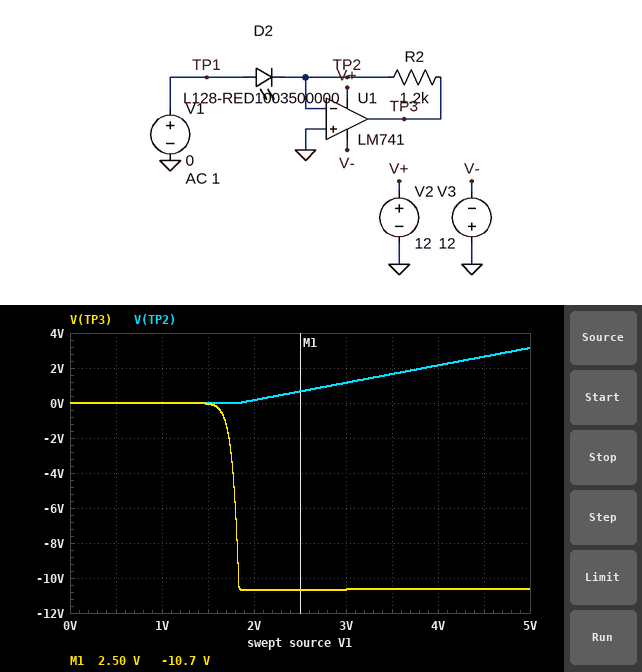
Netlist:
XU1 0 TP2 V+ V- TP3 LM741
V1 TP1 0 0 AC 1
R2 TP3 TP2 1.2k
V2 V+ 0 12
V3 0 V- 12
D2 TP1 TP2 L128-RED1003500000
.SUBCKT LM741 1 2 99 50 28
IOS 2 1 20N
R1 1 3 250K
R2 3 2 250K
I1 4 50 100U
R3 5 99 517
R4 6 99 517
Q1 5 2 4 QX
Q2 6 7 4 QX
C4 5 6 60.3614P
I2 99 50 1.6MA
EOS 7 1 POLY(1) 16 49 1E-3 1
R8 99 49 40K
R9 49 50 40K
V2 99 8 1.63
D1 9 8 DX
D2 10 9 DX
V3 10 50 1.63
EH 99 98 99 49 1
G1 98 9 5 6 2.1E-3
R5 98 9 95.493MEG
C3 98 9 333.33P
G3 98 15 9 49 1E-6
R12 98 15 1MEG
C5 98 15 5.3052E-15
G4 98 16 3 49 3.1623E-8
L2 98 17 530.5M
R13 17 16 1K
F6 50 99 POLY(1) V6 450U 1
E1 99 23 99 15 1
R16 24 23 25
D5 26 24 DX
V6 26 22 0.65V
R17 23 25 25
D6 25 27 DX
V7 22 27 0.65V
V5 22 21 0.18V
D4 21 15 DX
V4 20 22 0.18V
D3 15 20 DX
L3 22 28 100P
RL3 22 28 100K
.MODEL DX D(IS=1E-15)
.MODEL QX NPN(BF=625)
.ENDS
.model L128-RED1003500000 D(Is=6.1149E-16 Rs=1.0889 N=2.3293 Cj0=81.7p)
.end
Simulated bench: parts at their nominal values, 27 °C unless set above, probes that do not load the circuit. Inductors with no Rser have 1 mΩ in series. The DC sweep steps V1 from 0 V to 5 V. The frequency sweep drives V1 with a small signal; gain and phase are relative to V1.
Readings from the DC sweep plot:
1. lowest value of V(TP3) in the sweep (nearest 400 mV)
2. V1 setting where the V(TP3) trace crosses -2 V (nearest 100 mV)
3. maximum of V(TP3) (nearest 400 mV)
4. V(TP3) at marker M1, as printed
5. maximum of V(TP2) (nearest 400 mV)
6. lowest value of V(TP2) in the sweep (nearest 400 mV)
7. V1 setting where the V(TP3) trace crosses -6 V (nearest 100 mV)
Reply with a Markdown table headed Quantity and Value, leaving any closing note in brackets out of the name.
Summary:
| Quantity | Value |
|---|---|
| lowest value of V(TP3) in the sweep | -10.8 V |
| V1 setting where the V(TP3) trace crosses -2 V | 1.7 V |
| maximum of V(TP3) | 0 V |
| V(TP3) at marker M1, as printed | -10.7 V |
| maximum of V(TP2) | 3.2 V |
| lowest value of V(TP2) in the sweep | 0 V |
| V1 setting where the V(TP3) trace crosses -6 V | 1.8 V |
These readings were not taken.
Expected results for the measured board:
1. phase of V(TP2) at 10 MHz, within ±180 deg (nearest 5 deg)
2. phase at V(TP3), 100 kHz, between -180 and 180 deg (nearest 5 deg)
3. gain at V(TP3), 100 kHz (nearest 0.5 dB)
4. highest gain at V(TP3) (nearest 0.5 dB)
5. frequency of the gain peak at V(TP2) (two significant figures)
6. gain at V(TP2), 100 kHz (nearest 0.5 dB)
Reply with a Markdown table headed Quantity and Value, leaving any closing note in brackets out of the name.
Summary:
| Quantity | Value |
|---|---|
| phase of V(TP2) at 10 MHz, within ±180 deg | 10 deg |
| phase at V(TP3), 100 kHz, between -180 and 180 deg | -95 deg |
| gain at V(TP3), 100 kHz | -24.0 dB |
| highest gain at V(TP3) | 0.5 dB |
| frequency of the gain peak at V(TP2) | 1.2 MHz |
| gain at V(TP2), 100 kHz | -43.0 dB |
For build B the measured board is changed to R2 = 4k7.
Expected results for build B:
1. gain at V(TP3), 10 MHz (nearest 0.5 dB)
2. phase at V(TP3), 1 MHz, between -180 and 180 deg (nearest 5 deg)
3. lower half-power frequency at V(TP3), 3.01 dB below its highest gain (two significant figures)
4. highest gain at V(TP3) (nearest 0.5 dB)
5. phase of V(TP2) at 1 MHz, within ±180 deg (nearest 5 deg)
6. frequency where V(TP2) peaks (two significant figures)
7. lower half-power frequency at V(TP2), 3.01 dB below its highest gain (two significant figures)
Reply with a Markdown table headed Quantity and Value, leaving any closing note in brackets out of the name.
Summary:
| Quantity | Value |
|---|---|
| gain at V(TP3), 10 MHz | -24.5 dB |
| phase at V(TP3), 1 MHz, between -180 and 180 deg | 80 deg |
| lower half-power frequency at V(TP3), 3.01 dB below its highest gain | 510 kHz |
| highest gain at V(TP3) | 12.5 dB |
| phase of V(TP2) at 1 MHz, within ±180 deg | 20 deg |
| frequency where V(TP2) peaks | 630 kHz |
| lower half-power frequency at V(TP2), 3.01 dB below its highest gain | 540 kHz |
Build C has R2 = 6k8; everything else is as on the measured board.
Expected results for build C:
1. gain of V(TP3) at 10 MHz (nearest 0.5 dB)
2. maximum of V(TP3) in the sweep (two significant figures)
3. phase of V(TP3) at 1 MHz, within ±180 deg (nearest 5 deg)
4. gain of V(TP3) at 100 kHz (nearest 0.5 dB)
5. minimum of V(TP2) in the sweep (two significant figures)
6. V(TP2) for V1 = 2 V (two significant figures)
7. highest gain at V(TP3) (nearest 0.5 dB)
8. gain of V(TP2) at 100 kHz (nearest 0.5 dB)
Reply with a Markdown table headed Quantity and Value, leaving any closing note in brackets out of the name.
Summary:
| Quantity | Value |
|---|---|
| gain of V(TP3) at 10 MHz | -26.0 dB |
| maximum of V(TP3) in the sweep | 1.7 mV |
| phase of V(TP3) at 1 MHz, within ±180 deg | 75 deg |
| gain of V(TP3) at 100 kHz | -9.0 dB |
| minimum of V(TP2) in the sweep | 1.0 mV |
| V(TP2) for V1 = 2 V | 270 mV |
| highest gain at V(TP3) | 15.5 dB |
| gain of V(TP2) at 100 kHz | -28.5 dB |
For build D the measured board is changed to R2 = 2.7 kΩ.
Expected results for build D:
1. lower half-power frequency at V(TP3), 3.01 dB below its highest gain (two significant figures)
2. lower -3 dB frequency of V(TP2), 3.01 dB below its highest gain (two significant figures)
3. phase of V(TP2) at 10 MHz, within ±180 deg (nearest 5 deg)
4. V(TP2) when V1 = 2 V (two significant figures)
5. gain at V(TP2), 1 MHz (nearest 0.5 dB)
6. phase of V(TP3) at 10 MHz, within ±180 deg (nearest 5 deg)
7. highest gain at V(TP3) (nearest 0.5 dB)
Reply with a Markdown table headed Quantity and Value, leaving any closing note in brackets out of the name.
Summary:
| Quantity | Value |
|---|---|
| lower half-power frequency at V(TP3), 3.01 dB below its highest gain | 620 kHz |
| lower -3 dB frequency of V(TP2), 3.01 dB below its highest gain | 670 kHz |
| phase of V(TP2) at 10 MHz, within ±180 deg | 5 deg |
| V(TP2) when V1 = 2 V | 220 mV |
| gain at V(TP2), 1 MHz | 4.5 dB |
| phase of V(TP3) at 10 MHz, within ±180 deg | -5 deg |
| highest gain at V(TP3) | 7.5 dB |
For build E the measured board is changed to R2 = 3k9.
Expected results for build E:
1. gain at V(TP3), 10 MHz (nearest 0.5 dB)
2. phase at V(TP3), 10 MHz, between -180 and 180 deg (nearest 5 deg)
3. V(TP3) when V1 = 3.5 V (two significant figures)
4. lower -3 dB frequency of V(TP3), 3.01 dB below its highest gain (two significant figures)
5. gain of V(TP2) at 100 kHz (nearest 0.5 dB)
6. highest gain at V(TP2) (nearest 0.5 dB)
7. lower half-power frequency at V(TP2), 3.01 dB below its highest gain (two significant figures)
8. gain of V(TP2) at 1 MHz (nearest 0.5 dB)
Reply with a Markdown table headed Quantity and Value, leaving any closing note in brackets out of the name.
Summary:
| Quantity | Value |
|---|---|
| gain at V(TP3), 10 MHz | -23.5 dB |
| phase at V(TP3), 10 MHz, between -180 and 180 deg | -10 deg |
| V(TP3) when V1 = 3.5 V | -11 V |
| lower -3 dB frequency of V(TP3), 3.01 dB below its highest gain | 550 kHz |
| gain of V(TP2) at 100 kHz | -33.5 dB |
| highest gain at V(TP2) | 8.0 dB |
| lower half-power frequency at V(TP2), 3.01 dB below its highest gain | 580 kHz |
| gain of V(TP2) at 1 MHz | 3.5 dB |
